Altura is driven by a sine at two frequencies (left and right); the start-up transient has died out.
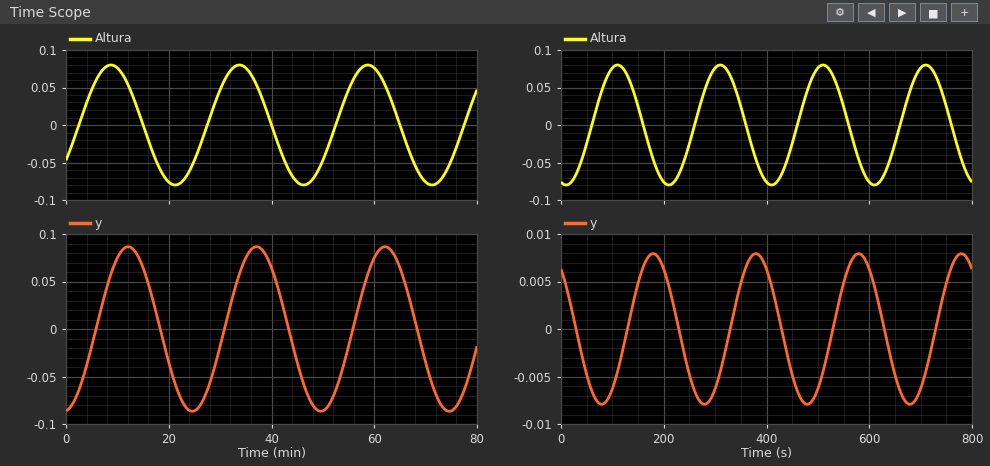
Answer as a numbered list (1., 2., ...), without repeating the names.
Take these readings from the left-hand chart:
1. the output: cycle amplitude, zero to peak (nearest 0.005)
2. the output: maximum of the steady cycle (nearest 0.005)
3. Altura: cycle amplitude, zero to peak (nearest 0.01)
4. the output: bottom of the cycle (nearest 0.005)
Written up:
1. 0.085
2. 0.085
3. 0.08
4. -0.085
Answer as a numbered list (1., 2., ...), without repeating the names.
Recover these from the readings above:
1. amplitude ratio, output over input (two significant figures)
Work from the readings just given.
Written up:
1. 1.1
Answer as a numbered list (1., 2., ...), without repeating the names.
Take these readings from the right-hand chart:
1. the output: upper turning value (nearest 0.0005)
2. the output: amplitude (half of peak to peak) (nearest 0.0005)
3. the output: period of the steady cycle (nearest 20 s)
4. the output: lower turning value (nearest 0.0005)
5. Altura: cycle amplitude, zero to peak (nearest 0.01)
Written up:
1. 0.0080
2. 0.0080
3. 200 s
4. -0.0080
5. 0.08
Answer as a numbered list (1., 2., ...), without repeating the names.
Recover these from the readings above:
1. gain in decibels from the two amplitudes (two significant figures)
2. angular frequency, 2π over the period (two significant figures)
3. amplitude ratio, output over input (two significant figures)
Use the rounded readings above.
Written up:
1. -20 dB
2. 0.031 rad/s
3. 0.10
